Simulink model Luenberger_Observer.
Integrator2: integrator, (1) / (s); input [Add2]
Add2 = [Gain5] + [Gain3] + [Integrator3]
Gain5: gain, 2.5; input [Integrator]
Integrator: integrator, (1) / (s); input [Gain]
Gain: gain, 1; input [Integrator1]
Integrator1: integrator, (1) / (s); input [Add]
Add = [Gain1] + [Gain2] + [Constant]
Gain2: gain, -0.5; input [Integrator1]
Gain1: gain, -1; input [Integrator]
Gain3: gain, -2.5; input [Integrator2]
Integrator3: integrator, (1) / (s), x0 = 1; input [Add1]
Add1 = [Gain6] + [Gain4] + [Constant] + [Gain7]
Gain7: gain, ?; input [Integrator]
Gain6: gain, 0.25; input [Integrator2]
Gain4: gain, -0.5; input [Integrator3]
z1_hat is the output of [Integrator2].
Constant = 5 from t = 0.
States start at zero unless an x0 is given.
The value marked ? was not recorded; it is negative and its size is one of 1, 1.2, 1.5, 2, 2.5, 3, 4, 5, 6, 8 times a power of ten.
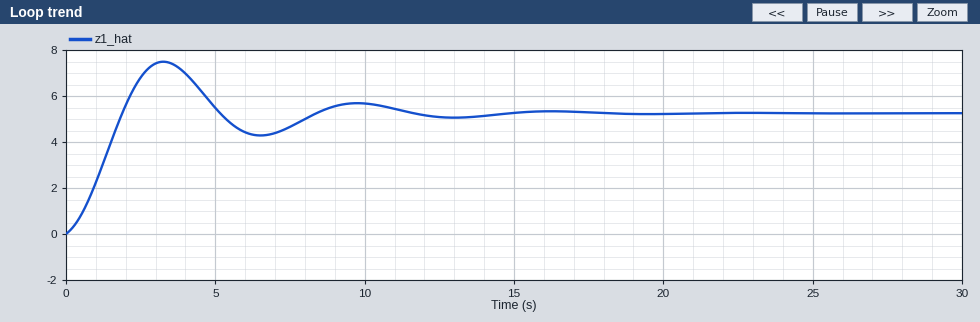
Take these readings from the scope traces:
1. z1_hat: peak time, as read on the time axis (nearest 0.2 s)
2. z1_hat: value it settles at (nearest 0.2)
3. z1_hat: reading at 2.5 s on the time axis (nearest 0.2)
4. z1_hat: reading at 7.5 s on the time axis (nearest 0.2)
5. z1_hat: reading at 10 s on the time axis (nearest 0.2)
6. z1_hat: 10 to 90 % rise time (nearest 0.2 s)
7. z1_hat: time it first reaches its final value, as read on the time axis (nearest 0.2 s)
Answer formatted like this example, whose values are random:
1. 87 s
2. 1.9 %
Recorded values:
1. 3.2 s
2. 5.2
3. 6.8
4. 4.6
5. 5.6
6. 1.4 s
7. 1.8 s
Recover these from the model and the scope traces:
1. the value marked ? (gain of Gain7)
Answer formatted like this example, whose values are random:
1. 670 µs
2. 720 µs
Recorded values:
1. -1.2
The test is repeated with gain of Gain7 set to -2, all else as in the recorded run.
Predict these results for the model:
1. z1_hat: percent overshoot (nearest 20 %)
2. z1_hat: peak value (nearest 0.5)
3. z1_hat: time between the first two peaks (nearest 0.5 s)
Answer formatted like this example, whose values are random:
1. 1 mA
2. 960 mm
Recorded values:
1. 340 %
2. 5.5
3. 6.5 s
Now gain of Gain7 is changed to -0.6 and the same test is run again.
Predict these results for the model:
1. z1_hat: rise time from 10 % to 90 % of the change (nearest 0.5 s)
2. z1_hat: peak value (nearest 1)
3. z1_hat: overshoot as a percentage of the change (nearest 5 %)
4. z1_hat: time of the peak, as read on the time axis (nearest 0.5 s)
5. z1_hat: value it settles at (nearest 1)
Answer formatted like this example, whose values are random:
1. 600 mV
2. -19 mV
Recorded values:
1. 2.0 s
2. 9
3. 15 %
4. 3.5 s
5. 8
